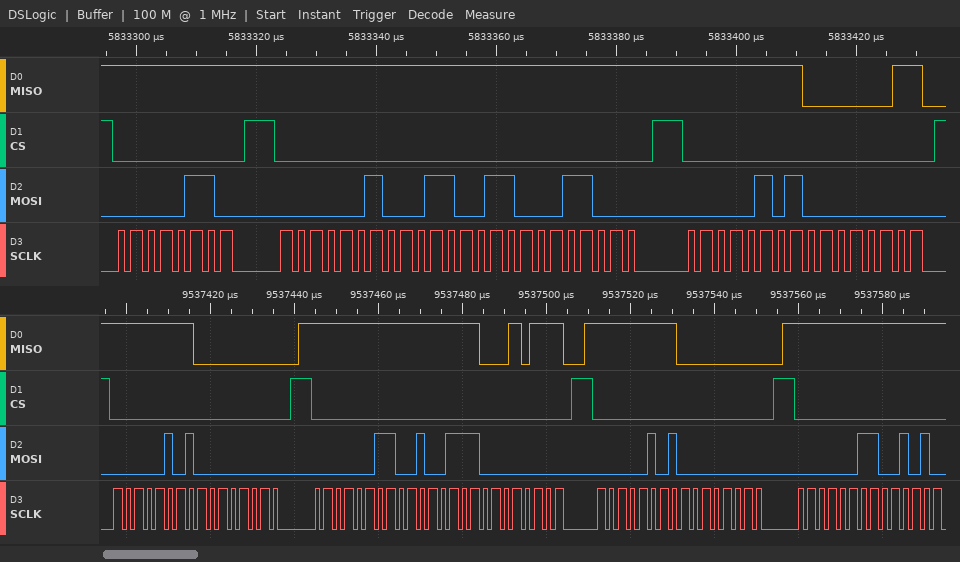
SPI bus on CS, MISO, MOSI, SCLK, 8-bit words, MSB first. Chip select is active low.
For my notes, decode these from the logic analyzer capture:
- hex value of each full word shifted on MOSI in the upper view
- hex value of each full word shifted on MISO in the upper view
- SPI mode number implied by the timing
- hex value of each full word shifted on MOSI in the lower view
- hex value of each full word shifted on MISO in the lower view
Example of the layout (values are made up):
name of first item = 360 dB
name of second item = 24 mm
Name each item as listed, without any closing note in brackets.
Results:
hex value of each full word shifted on MOSI in the upper view = 06, 02, 33, 18, 05, 00
hex value of each full word shifted on MISO in the upper view = FF, FF, FF, FF, FF, 03
SPI mode number implied by the timing = 0
hex value of each full word shifted on MOSI in the lower view = 05, 00, 03, 27, 00, 05, 00, 03
hex value of each full word shifted on MISO in the lower view = FF, 00, FF, FF, 17, FF, 00, FF
